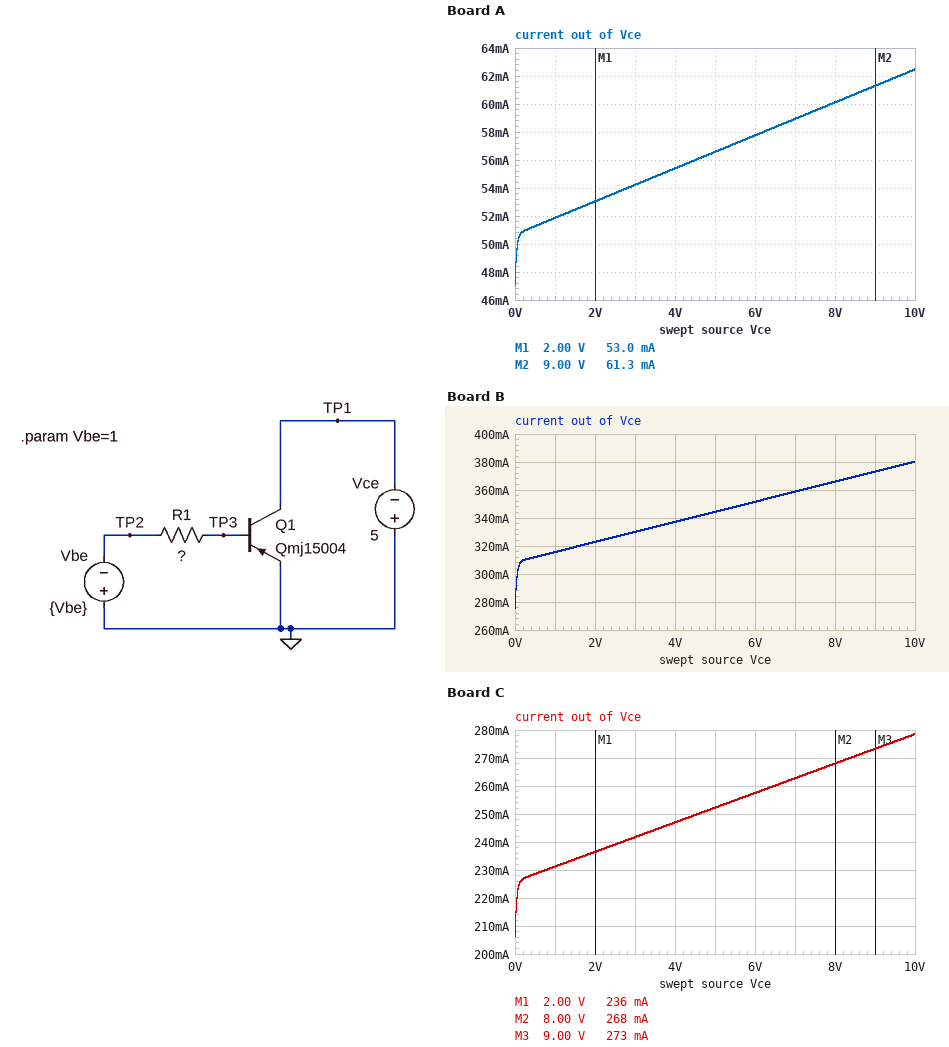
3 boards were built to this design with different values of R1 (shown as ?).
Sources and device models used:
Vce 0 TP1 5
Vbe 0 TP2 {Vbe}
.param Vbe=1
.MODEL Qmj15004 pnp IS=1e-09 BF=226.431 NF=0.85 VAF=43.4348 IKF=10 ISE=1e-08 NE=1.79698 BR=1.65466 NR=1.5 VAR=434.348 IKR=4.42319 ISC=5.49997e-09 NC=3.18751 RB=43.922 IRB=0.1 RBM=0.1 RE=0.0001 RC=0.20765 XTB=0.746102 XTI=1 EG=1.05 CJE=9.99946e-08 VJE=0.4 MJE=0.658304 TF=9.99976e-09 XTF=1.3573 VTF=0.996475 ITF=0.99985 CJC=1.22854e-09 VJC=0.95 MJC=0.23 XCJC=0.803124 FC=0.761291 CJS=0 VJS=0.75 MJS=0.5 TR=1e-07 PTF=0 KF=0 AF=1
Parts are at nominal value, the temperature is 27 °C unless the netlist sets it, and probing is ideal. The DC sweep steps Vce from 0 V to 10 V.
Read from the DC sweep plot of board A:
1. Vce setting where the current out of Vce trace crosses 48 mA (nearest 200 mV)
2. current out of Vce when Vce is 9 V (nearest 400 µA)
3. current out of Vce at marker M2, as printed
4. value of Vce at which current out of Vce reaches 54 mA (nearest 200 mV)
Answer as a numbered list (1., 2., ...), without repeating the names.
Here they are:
1. 0 V
2. 61.2 mA
3. 61.3 mA
4. 2.8 V
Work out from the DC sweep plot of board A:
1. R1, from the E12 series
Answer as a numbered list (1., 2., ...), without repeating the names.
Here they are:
1. 2.2 kΩ
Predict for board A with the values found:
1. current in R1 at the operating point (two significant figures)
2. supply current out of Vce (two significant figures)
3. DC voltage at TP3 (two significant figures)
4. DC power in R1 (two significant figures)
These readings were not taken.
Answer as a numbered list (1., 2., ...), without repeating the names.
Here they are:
1. 270 µA
2. 57 mA
3. -400 mV
4. 160 µW
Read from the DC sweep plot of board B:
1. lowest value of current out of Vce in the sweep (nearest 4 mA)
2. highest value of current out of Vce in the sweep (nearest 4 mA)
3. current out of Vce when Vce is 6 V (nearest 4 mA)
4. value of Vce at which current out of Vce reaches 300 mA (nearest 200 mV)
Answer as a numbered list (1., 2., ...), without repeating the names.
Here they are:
1. 276 mA
2. 380 mA
3. 352 mA
4. 0 V
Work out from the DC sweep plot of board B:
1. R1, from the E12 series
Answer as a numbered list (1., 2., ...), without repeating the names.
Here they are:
1. 330 Ω
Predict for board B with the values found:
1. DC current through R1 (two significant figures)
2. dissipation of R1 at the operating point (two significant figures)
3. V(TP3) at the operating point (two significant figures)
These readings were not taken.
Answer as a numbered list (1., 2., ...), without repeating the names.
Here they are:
1. 1.5 mA
2. 770 µW
3. -500 mV
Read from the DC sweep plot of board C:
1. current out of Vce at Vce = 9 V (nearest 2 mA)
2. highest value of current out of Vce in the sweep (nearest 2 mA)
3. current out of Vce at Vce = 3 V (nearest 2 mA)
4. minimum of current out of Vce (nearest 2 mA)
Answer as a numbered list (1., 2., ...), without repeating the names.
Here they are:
1. 274 mA
2. 278 mA
3. 242 mA
4. 206 mA
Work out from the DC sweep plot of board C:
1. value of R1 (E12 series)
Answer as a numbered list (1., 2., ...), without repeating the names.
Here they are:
1. 470 Ω
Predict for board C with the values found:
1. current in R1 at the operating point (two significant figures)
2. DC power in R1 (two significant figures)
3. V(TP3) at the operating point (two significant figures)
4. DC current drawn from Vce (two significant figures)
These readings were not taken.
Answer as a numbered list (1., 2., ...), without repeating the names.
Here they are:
1. 1.1 mA
2. 590 µW
3. -470 mV
4. 250 mA
